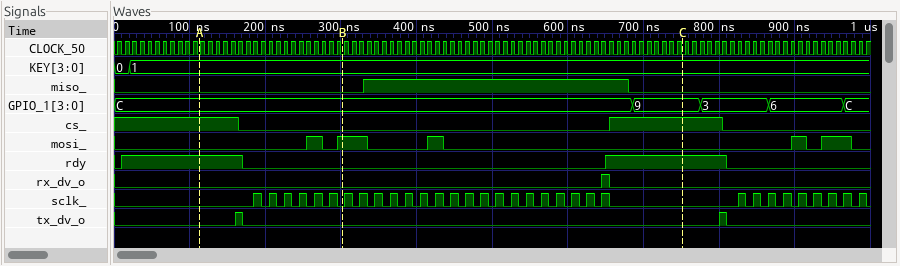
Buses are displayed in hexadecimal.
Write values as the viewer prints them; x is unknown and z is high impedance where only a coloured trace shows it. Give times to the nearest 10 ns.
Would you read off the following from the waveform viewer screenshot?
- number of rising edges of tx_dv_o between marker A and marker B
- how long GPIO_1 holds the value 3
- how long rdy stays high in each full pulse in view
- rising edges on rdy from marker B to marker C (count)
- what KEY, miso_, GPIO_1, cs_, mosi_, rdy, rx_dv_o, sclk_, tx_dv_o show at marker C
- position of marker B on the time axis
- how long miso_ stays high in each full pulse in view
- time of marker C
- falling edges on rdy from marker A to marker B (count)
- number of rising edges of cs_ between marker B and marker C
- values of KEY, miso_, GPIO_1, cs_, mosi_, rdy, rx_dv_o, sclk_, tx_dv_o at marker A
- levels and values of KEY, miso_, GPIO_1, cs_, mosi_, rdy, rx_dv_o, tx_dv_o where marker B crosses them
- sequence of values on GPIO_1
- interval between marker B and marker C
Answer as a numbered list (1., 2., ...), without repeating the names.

1. 1
2. 90 ns
3. 160 ns, 160 ns
4. 1
5. KEY=1, miso_=0, GPIO_1=9, cs_=1, mosi_=0, rdy=1, rx_dv_o=0, sclk_=0, tx_dv_o=0
6. 300 ns
7. 350 ns
8. 750 ns
9. 1
10. 1
11. KEY=1, miso_=0, GPIO_1=C, cs_=1, mosi_=0, rdy=1, rx_dv_o=0, sclk_=0, tx_dv_o=0
12. KEY=1, miso_=0, GPIO_1=C, cs_=0, mosi_=1, rdy=0, rx_dv_o=0, tx_dv_o=0
13. C, 9, 3, 6, C
14. 450 ns
